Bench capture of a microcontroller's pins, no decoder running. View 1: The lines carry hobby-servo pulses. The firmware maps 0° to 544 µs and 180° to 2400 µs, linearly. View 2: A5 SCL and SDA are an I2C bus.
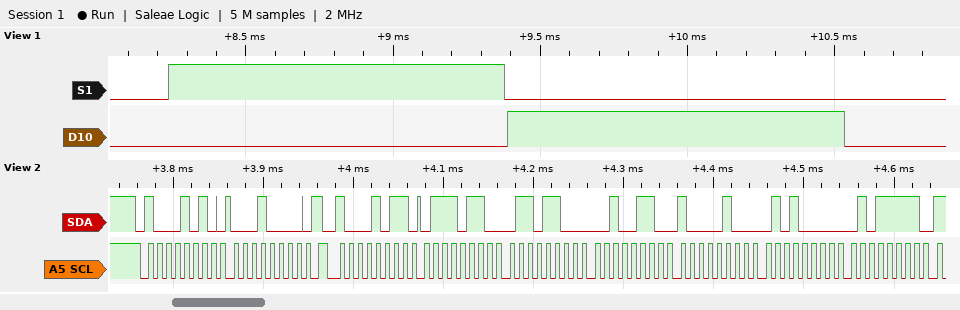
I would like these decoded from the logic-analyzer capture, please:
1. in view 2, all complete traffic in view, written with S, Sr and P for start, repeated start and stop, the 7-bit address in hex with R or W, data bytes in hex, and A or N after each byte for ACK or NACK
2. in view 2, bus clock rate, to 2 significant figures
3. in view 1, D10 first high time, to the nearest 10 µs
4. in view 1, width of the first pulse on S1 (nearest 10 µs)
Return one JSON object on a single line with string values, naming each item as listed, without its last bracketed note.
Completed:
{"in view 2, all complete traffic in view, written with S, Sr and P for start, repeated start and stop, the 7-bit address in hex with R or W, data bytes in hex, and A or N after each byte for ACK or NACK": "S 45W A 10 A Sr 45R A 76 A 6C A 26 A 84 A 50 A 5F A", "in view 2, bus clock rate, to 2 significant figures": "100 kHz", "in view 1, D10 first high time, to the nearest 10 µs": "1140 µs", "in view 1, width of the first pulse on S1": "1140 µs"}
